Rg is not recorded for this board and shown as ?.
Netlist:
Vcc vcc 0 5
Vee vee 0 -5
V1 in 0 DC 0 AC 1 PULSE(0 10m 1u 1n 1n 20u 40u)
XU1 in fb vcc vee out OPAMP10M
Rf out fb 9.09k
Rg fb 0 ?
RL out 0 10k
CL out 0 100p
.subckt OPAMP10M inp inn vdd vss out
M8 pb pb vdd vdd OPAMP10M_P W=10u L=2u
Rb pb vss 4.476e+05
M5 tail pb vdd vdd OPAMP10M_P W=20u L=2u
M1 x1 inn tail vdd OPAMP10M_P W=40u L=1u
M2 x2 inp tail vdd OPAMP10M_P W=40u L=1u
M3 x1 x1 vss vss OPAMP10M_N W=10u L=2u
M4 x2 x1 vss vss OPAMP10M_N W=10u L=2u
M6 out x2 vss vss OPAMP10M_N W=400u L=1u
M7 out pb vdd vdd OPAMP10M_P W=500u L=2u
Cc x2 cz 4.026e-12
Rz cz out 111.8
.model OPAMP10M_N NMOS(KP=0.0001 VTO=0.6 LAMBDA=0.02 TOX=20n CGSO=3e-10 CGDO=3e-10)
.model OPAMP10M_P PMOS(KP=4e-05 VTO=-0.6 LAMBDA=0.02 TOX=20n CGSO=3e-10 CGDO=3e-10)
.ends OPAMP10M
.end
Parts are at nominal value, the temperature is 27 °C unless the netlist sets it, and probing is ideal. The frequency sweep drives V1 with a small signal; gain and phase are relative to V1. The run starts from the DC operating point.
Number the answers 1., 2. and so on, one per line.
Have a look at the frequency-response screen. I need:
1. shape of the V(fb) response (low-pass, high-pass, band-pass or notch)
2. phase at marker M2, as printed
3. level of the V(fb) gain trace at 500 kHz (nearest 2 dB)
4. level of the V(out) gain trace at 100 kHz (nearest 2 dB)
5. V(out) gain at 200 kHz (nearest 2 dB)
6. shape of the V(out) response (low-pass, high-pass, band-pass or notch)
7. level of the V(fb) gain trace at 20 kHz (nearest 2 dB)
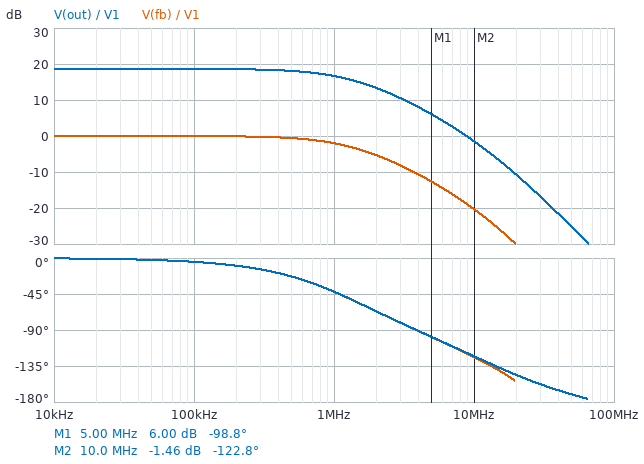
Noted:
1. low-pass
2. -122.8 deg
3. 0 dB
4. 18 dB
5. 18 dB
6. low-pass
7. 0 dB
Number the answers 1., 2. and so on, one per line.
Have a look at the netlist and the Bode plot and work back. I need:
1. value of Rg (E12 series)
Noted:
1. 1.2 kΩ
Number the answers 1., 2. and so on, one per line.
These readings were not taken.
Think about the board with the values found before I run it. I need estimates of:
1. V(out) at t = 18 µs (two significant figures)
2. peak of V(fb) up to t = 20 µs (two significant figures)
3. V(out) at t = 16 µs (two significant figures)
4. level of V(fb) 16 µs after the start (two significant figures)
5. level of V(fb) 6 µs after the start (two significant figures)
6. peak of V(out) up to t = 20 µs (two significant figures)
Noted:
1. 84 mV
2. 9.8 mV
3. 84 mV
4. 9.8 mV
5. 9.8 mV
6. 84 mV
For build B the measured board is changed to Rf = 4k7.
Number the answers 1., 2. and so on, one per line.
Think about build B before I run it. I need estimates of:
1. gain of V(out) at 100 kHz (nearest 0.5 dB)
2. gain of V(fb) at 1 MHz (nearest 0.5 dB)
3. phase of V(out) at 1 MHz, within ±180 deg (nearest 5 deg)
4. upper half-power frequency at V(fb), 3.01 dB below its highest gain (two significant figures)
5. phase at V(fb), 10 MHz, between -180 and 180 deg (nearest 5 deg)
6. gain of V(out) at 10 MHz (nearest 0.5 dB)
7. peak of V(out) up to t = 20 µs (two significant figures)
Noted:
1. 14.0 dB
2. -0.5 dB
3. -25 deg
4. 2.4 MHz
5. -120 deg
6. -1.0 dB
7. 48 mV
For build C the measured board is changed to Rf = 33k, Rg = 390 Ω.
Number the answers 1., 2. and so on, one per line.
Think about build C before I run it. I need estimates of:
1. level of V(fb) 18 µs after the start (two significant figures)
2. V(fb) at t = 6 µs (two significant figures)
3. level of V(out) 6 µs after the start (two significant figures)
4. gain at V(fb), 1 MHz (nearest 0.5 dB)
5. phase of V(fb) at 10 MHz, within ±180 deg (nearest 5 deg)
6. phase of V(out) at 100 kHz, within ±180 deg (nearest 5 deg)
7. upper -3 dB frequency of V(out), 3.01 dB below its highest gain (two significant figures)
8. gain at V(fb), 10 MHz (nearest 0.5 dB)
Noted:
1. 9.8 mV
2. 9.5 mV
3. 820 mV
4. -18.5 dB
5. -130 deg
6. -40 deg
7. 120 kHz
8. -41.0 dB
